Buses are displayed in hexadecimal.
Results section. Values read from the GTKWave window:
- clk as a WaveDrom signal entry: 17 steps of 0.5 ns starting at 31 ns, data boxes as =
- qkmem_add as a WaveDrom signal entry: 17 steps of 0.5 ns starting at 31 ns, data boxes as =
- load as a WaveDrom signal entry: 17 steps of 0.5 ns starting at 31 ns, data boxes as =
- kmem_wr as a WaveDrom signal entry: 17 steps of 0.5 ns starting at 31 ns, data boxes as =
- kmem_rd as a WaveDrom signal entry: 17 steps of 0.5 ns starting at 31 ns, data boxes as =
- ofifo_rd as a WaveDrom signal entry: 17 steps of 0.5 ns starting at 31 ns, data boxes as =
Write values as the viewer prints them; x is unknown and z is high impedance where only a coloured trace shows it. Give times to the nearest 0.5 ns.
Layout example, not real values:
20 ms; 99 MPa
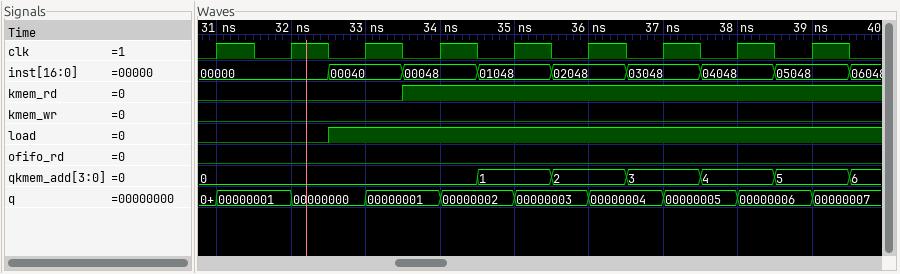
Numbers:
{name: 'clk', wave: '10101010101010101'}; {name: 'qkmem_add', wave: '=......=.=.=.=.=.', data: '0 1 2 3 4 5'}; {name: 'load', wave: '0..1.............'}; {name: 'kmem_wr', wave: '0................'}; {name: 'kmem_rd', wave: '0....1...........'}; {name: 'ofifo_rd', wave: '0................'}
